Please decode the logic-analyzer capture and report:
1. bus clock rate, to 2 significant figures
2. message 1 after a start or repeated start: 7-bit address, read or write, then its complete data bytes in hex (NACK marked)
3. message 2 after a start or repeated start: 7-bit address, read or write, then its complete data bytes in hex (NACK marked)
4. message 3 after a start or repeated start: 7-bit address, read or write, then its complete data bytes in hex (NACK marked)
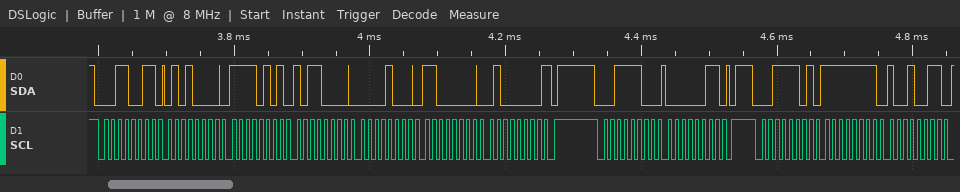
100 kHz
0x19 read: 50 F5 B0 08 C0 40 NACK
0x1E write: 03
0x1E read: FF 93
